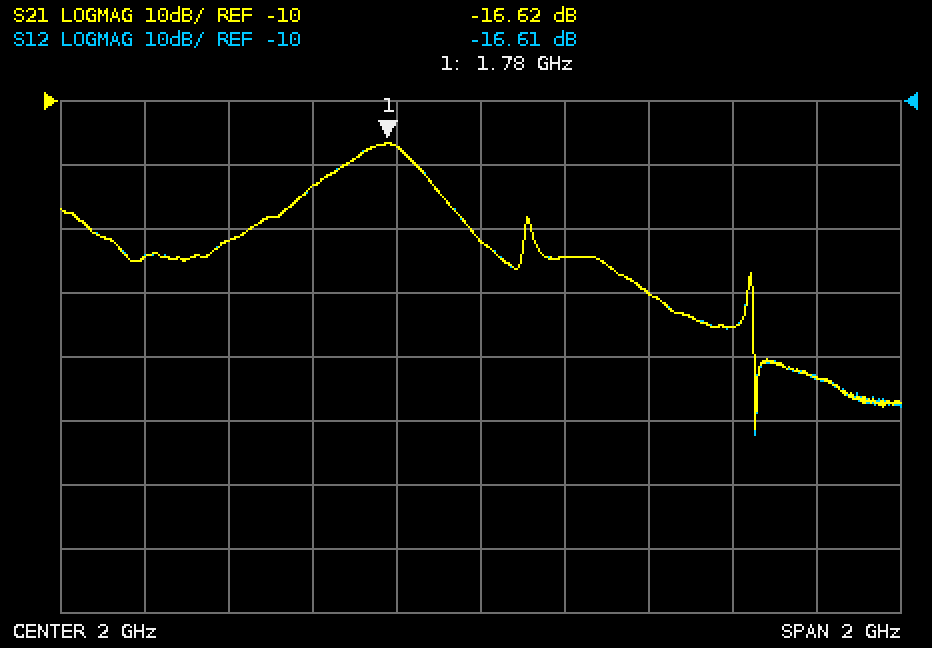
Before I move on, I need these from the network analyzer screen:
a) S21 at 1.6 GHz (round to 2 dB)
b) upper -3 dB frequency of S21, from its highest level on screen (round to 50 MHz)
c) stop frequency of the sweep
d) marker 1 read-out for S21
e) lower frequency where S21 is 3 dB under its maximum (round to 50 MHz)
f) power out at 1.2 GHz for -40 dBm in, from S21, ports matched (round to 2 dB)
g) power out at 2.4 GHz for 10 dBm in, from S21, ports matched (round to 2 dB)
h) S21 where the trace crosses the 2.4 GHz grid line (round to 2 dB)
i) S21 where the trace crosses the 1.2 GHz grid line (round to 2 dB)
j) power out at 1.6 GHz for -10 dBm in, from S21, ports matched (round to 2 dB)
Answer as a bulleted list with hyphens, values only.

- -24 dB
- 1.85 GHz
- 3 GHz
- -16.62 dB
- 1.70 GHz
- -74 dBm
- -30 dBm
- -40 dB
- -34 dB
- -34 dBm
